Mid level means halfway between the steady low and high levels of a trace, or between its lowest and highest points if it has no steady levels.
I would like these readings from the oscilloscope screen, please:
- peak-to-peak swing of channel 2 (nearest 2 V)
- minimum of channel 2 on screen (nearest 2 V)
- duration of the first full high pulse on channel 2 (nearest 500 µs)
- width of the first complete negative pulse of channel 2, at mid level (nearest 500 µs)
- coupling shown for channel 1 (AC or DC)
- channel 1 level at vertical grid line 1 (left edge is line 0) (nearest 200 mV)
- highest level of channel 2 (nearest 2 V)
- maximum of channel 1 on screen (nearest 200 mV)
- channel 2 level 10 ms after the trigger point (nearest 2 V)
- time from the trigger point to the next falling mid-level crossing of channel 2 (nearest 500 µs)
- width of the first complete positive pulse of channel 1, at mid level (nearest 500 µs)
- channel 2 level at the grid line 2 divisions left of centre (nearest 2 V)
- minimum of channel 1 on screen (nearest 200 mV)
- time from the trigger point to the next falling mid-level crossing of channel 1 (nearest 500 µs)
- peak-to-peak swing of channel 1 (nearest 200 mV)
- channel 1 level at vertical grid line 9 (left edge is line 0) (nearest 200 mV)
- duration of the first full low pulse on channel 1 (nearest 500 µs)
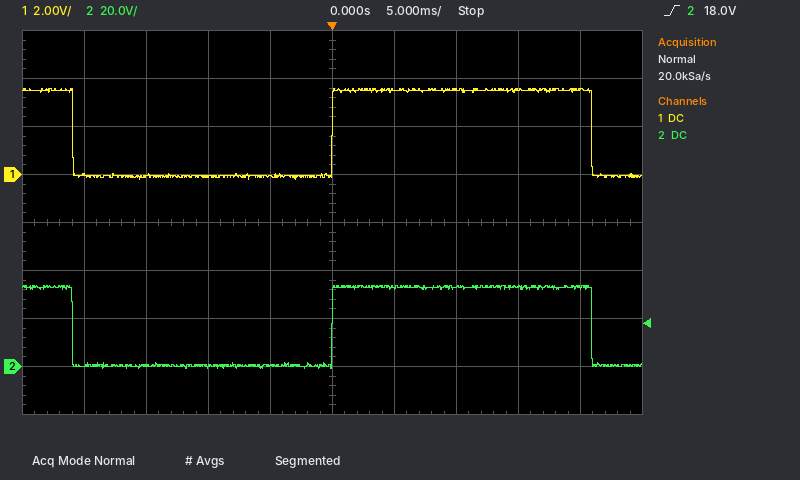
34 V
0 V
21.0 ms
21.0 ms
DC
0.0 V
34 V
3.6 V
34 V
21.0 ms
21.0 ms
0 V
-200 mV
21.0 ms
3.8 V
3.6 V
21.0 ms
